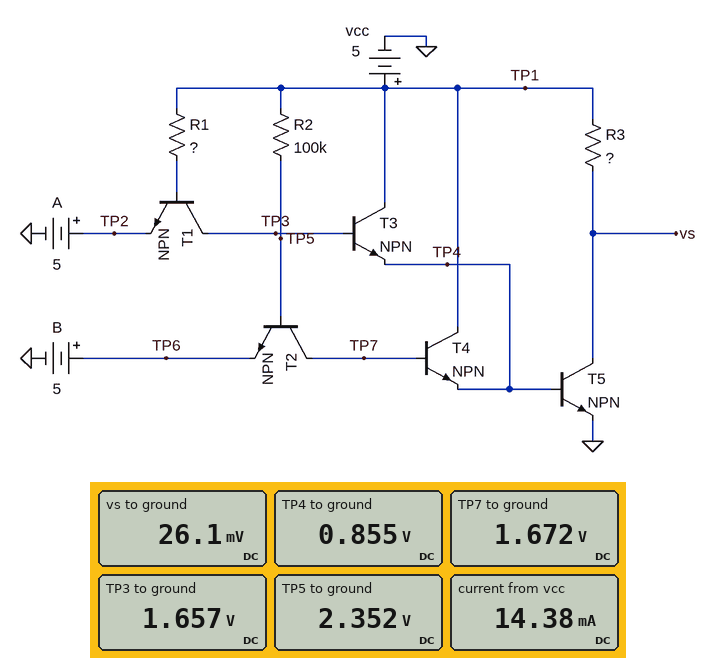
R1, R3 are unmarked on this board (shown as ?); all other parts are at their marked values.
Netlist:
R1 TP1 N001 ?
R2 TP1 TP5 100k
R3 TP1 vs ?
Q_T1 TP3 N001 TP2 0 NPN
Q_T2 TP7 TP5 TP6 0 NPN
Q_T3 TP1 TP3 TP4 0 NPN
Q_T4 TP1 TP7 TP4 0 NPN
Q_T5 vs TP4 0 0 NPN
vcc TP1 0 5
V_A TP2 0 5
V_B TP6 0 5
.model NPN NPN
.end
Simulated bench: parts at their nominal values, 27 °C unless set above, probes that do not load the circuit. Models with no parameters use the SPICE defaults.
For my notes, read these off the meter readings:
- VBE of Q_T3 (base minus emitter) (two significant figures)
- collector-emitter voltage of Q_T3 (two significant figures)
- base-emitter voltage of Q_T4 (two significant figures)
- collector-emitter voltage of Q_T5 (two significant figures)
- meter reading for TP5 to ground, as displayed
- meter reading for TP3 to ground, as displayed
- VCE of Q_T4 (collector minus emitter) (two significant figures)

800 mV
4.1 V
820 mV
26 mV
2.352 V
1.657 V
4.1 V
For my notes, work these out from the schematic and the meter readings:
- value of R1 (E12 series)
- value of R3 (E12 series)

180 kΩ
820 Ω
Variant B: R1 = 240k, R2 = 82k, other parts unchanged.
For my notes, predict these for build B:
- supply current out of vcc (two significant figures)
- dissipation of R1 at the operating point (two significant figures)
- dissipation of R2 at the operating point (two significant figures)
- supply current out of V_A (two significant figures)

15 mA
30 µW
85 µW
11 µA
